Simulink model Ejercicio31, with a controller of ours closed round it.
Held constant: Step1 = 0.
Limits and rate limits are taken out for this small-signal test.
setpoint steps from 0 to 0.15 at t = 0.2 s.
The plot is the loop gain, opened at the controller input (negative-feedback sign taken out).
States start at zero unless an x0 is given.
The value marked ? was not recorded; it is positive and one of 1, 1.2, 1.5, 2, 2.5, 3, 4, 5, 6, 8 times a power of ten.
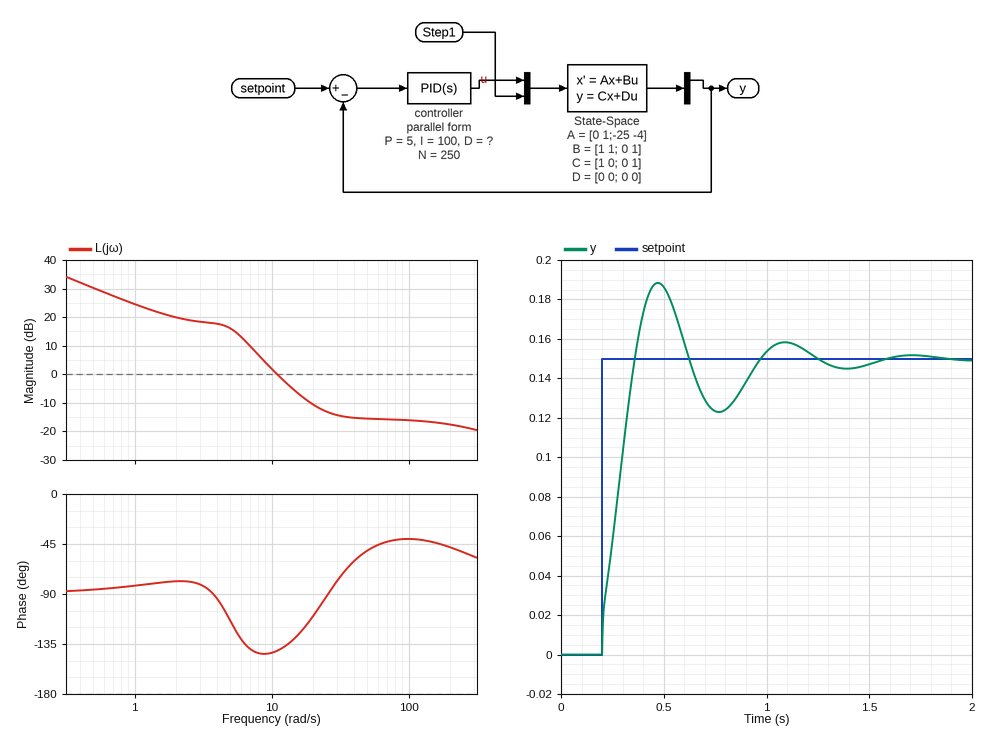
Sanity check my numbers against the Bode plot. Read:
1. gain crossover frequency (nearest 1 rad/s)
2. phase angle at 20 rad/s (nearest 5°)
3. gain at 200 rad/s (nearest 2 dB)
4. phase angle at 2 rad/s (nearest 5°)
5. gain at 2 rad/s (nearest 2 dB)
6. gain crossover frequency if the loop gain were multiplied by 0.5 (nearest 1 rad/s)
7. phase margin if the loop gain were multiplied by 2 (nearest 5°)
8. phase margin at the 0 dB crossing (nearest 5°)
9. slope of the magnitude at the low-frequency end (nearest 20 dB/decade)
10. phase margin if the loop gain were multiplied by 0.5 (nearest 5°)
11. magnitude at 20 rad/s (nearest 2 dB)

11 rad/s
-110°
-18 dB
-80°
20 dB
8 rad/s
50°
40°
-20 dB/decade
35°
-10 dB
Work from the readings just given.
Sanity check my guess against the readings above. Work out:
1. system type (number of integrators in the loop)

1
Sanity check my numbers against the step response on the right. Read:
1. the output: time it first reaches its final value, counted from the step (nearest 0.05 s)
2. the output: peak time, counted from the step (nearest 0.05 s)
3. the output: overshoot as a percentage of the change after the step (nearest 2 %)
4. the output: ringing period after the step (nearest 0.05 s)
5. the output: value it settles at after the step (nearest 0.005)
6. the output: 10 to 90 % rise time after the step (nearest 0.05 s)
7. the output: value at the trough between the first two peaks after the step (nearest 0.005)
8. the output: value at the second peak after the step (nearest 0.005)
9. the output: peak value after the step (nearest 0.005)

0.15 s
0.25 s
26 %
0.60 s
0.150
0.15 s
0.125
0.160
0.190
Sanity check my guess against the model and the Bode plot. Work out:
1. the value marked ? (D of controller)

0.15
